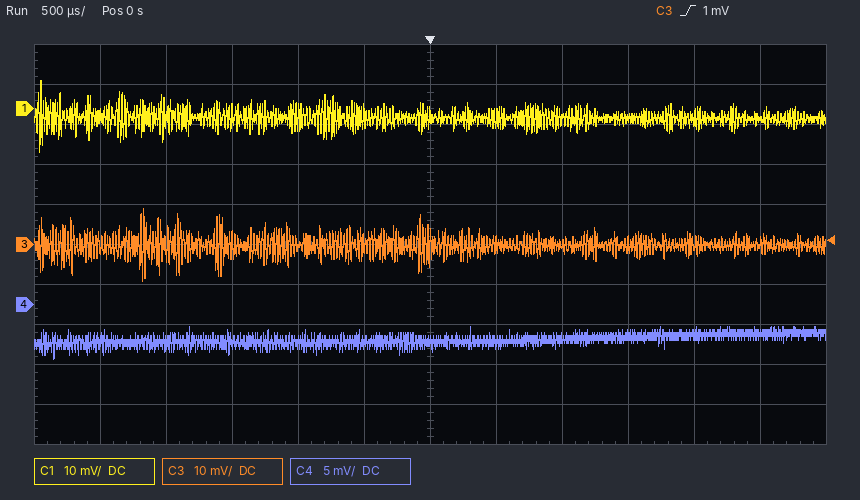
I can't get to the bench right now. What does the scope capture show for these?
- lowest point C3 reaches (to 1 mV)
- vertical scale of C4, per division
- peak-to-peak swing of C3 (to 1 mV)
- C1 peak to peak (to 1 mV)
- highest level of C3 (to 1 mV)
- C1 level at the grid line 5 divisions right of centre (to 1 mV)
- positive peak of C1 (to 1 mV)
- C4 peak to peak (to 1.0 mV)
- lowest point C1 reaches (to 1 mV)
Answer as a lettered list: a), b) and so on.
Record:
a) -9 mV
b) 5 mV
c) 18 mV
d) 18 mV
e) 9 mV
f) -2 mV
g) 7 mV
h) 4.0 mV
i) -11 mV
